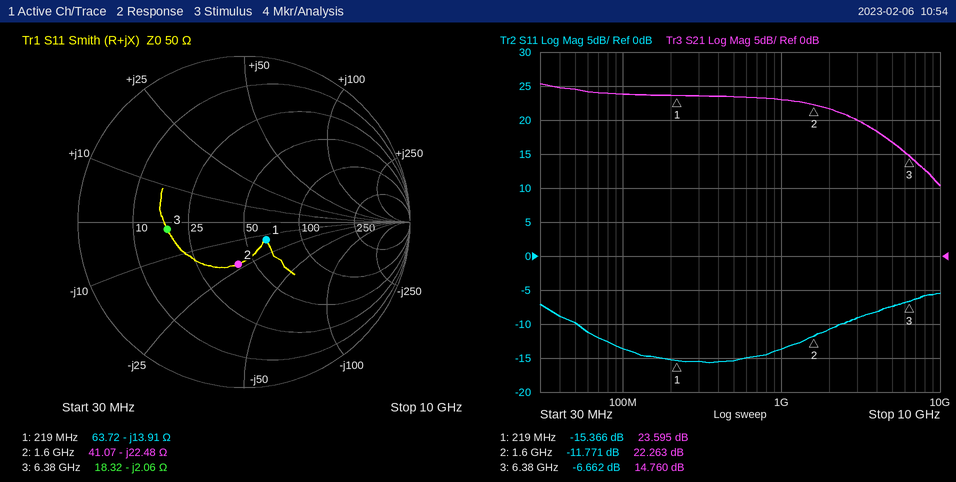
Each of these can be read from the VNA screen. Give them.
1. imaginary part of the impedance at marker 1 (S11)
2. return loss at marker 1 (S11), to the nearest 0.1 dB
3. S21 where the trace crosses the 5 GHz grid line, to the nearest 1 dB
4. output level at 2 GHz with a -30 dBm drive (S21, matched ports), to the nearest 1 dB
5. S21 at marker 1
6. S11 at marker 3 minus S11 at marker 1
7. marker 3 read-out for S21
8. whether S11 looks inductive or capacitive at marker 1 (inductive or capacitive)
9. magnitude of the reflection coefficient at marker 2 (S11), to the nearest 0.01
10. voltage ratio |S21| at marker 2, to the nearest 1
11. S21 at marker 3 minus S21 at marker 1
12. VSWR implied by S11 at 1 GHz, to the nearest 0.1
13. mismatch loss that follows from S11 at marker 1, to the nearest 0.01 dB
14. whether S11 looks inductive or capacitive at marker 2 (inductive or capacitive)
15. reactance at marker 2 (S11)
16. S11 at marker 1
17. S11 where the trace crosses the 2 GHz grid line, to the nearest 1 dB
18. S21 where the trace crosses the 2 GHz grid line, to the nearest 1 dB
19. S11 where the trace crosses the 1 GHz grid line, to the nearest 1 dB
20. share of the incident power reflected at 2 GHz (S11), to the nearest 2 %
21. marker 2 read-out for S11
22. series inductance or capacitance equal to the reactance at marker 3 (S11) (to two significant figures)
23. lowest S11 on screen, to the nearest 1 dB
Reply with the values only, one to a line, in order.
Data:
-13.91 Ω
15.4 dB
17 dB
-8 dBm
23.595 dB
8.704 dB
14.760 dB
capacitive
0.26
13
-8.835 dB
1.5
0.13 dB
capacitive
-22.48 Ω
-15.366 dB
-11 dB
22 dB
-14 dB
8 %
-11.771 dB
12 pF
-16 dB
